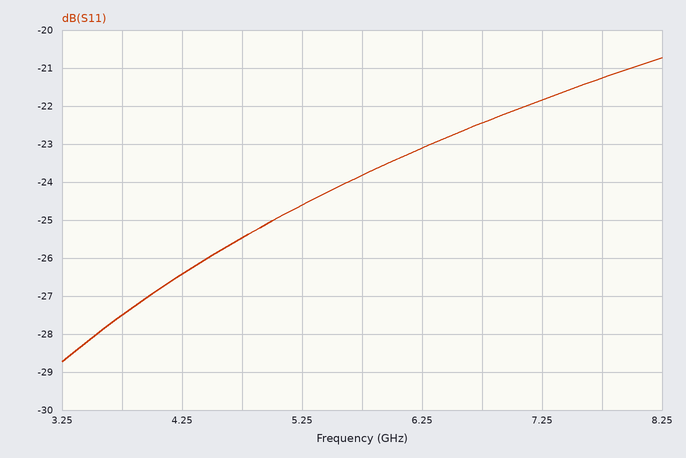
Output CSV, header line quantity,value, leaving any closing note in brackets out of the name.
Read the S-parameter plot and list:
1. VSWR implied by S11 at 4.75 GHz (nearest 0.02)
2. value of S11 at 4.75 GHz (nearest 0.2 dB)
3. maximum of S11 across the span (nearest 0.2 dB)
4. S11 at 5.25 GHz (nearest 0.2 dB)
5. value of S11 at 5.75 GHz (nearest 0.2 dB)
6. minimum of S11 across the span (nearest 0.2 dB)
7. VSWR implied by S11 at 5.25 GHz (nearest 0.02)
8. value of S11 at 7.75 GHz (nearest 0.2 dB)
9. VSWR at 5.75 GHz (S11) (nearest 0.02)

quantity,value
VSWR implied by S11 at 4.75 GHz,1.12
value of S11 at 4.75 GHz,-25.4 dB
maximum of S11 across the span,-20.8 dB
S11 at 5.25 GHz,-24.6 dB
value of S11 at 5.75 GHz,-23.8 dB
minimum of S11 across the span,-28.8 dB
VSWR implied by S11 at 5.25 GHz,1.12
value of S11 at 7.75 GHz,-21.2 dB
VSWR at 5.75 GHz (S11),1.14
